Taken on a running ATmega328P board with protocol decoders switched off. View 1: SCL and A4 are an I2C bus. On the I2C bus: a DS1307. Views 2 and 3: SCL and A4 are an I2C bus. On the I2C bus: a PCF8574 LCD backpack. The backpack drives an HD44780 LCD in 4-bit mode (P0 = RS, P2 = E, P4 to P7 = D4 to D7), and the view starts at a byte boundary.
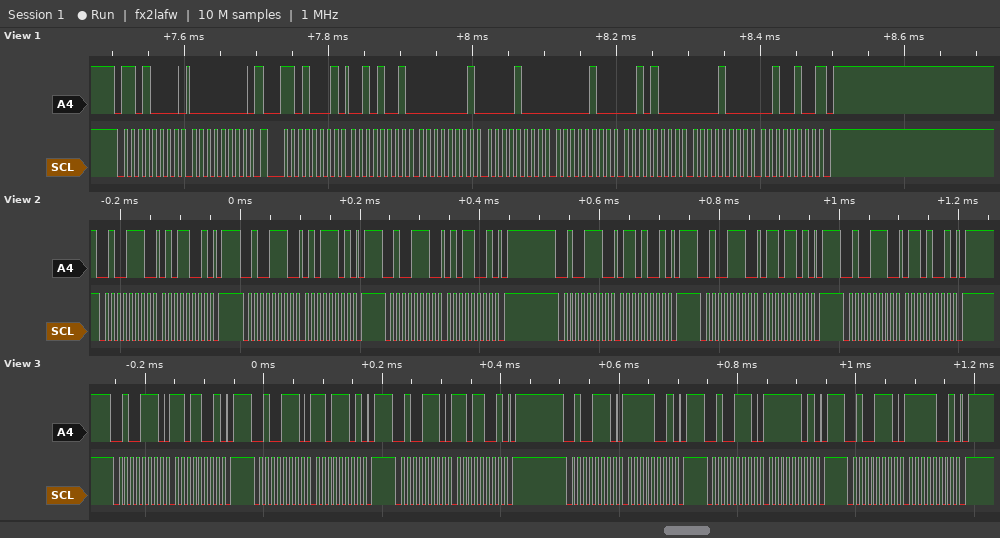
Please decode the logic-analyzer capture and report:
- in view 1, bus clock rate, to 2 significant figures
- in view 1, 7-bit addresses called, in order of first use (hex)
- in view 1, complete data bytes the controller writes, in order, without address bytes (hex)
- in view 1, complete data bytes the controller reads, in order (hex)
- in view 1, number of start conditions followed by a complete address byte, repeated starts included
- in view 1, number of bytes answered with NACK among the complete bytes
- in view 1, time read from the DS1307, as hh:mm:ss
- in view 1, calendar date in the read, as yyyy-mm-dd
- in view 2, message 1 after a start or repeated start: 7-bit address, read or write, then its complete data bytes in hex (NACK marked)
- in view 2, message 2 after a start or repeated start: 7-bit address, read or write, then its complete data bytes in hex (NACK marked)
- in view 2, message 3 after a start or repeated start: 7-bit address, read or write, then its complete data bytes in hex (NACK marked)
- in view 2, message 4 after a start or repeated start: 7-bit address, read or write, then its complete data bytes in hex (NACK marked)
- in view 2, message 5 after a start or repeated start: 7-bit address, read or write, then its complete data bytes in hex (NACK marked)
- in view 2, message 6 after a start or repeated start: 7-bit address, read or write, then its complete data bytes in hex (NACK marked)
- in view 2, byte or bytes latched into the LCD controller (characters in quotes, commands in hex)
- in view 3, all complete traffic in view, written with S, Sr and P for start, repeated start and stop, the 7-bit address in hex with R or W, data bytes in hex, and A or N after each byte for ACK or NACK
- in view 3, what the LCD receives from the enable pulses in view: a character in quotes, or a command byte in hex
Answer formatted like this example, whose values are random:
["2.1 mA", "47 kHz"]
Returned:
["100 kHz", "0x68", "00", "29 01 08 04 28 08 24", "2", "1", "08:01:29", "2024-08-28", "0x27 write: 59", "0x27 write: 5D", "0x27 write: 59", "0x27 write: 69", "0x27 write: 6D", "0x27 write: 69", "'V'", "S 27W A D9 A P S 27W A DD A P S 27W A D9 A P S 27W A F9 A P S 27W A FD A P S 27W A F9 A P", "data 0xDF"]
